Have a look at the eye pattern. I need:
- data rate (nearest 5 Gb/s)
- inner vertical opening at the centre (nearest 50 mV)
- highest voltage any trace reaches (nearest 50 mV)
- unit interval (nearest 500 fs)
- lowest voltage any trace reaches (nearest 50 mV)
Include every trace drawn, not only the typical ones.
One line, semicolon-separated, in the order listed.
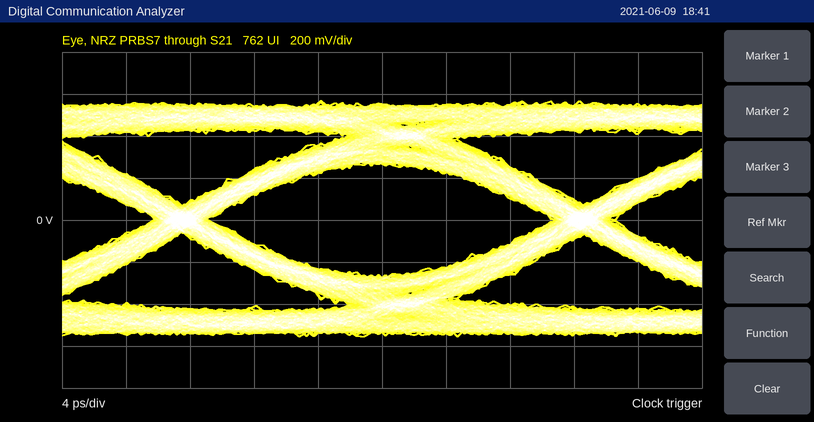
40 Gb/s; 550 mV; 550 mV; 25.0 ps; -550 mV
